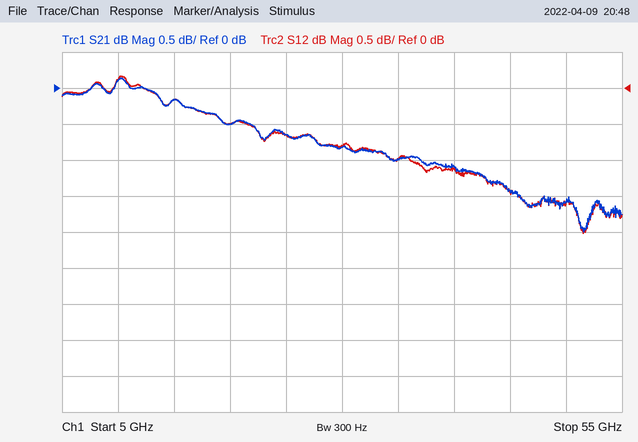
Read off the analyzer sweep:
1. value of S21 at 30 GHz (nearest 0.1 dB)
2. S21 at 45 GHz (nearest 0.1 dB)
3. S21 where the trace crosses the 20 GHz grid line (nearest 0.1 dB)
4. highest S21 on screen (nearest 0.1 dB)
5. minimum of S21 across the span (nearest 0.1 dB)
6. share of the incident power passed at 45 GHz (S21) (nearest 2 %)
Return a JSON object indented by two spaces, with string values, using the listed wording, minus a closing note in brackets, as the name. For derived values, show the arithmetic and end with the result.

{
  "value of S21 at 30 GHz": "-0.8 dB",
  "S21 at 45 GHz": "-1.4 dB",
  "S21 where the trace crosses the 20 GHz grid line": "-0.5 dB",
  "highest S21 on screen": "0.1 dB",
  "minimum of S21 across the span": "-2.0 dB",
  "share of the incident power passed at 45 GHz (S21)": "10^(-1.4/10) ≈ 72 %"
}
